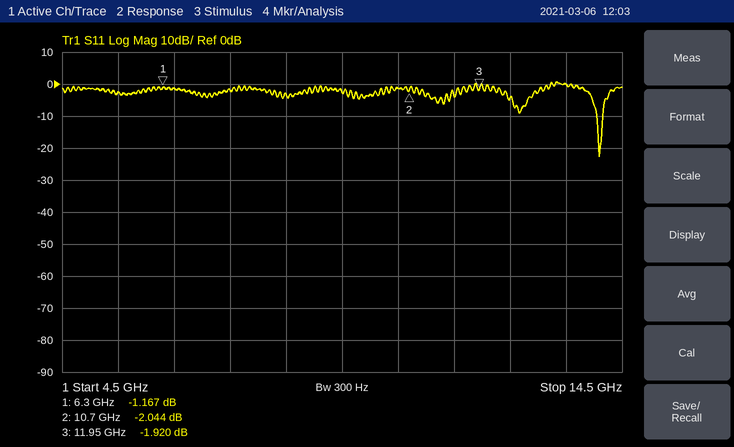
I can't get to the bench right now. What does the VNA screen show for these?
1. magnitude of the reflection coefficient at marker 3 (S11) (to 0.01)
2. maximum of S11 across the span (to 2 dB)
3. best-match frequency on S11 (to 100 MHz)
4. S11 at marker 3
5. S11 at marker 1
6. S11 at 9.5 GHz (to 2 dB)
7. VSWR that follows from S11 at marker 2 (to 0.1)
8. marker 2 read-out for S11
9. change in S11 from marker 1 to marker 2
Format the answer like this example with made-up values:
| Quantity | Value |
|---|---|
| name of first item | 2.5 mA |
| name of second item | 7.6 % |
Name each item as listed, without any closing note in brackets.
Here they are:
| Quantity | Value |
|---|---|
| magnitude of the reflection coefficient at marker 3 (S11) | 0.80 |
| maximum of S11 across the span | 0 dB |
| best-match frequency on S11 | 14.1 GHz |
| S11 at marker 3 | -1.920 dB |
| S11 at marker 1 | -1.167 dB |
| S11 at 9.5 GHz | -2 dB |
| VSWR that follows from S11 at marker 2 | 8.5 |
| marker 2 read-out for S11 | -2.044 dB |
| change in S11 from marker 1 to marker 2 | -0.877 dB |
